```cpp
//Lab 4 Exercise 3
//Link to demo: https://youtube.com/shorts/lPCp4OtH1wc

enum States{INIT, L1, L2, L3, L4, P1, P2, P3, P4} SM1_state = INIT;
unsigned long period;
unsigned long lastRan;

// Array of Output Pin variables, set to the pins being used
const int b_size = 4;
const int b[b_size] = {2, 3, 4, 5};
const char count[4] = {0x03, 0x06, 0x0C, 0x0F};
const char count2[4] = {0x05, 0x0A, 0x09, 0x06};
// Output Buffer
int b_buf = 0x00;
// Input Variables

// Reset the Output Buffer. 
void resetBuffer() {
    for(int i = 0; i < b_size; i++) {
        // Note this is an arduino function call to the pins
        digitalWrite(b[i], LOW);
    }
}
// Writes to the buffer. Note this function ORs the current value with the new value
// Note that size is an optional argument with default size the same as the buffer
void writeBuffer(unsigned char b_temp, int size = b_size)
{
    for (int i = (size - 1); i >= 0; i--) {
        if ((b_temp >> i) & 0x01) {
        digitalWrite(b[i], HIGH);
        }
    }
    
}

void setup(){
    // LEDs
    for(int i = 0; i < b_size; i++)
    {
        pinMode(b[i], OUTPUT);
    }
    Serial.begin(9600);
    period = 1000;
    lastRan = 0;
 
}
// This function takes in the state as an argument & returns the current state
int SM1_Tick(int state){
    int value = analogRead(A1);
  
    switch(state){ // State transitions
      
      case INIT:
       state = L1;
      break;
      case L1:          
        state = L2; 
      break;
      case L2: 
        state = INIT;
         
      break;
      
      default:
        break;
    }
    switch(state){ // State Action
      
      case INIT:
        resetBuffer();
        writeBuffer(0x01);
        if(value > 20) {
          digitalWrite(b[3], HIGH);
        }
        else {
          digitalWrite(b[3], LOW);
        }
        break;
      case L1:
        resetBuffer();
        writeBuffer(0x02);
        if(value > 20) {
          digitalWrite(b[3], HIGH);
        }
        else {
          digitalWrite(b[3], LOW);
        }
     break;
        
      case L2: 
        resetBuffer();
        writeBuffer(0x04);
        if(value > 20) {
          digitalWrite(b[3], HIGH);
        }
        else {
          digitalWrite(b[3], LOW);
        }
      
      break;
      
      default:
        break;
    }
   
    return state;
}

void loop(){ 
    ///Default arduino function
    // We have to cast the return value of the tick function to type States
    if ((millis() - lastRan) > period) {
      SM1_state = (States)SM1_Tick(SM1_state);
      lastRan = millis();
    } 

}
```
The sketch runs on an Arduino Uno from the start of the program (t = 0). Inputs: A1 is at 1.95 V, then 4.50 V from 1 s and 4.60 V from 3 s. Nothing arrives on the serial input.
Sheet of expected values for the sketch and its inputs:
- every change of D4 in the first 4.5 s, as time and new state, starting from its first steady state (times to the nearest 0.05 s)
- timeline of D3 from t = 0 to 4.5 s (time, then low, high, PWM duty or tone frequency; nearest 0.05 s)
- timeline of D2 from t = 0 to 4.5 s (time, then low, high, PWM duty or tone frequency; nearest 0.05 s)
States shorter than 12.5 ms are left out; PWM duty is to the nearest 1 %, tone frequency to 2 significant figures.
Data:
0 s low; 2 s high; 3 s low
0 s low; 1 s high; 2 s low; 4 s high
0 s low; 3 s high; 4 s low
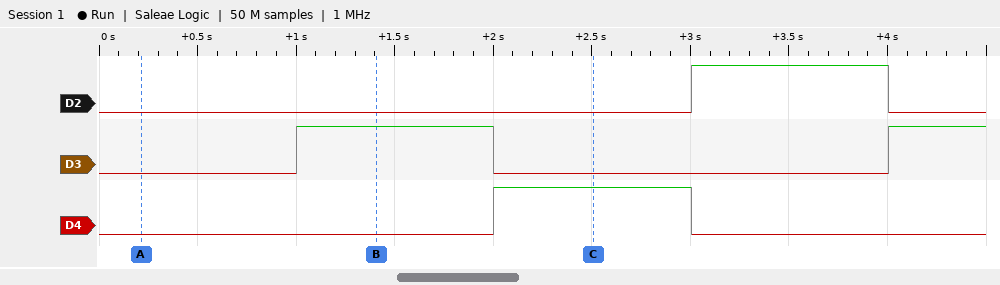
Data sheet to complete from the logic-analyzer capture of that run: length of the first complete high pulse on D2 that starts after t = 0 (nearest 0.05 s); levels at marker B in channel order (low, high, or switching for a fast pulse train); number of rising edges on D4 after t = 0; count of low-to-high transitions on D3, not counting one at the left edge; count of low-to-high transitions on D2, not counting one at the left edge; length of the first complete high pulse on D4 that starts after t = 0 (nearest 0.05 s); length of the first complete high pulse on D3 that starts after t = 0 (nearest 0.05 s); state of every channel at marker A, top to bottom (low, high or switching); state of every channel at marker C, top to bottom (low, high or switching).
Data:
1.00 s
D2 low, D3 high, D4 low
1
2
1
1.00 s
1.00 s
D2 low, D3 low, D4 low
D2 low, D3 low, D4 high
